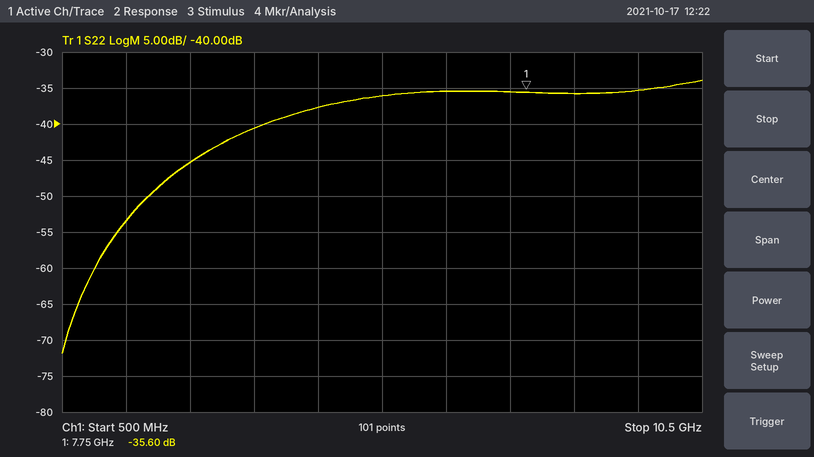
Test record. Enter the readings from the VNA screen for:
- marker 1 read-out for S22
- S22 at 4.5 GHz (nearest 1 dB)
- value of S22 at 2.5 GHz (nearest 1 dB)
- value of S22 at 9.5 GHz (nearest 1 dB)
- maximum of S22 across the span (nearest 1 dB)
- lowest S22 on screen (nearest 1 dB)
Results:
-35.60 dB
-38 dB
-45 dB
-35 dB
-34 dB
-72 dB
